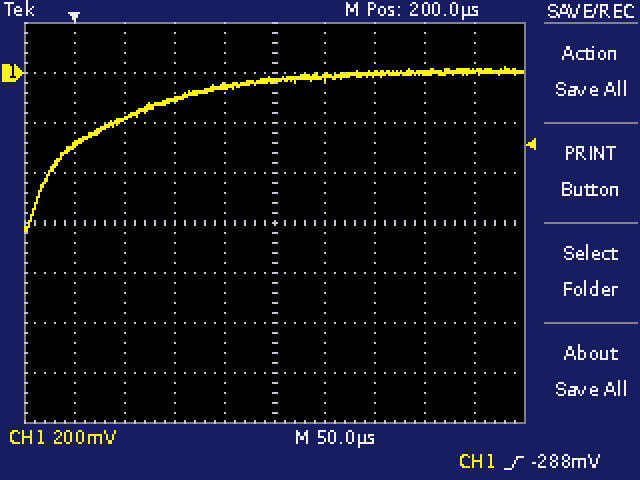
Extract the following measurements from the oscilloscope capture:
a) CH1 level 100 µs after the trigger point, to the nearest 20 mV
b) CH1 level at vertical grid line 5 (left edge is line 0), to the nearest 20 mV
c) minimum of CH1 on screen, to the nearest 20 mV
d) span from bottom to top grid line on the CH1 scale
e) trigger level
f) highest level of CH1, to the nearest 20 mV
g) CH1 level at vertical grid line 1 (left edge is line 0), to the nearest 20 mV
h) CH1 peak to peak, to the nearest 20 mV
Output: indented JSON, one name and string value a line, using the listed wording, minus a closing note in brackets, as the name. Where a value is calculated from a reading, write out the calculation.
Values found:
{
  "CH1 level 100 µs after the trigger point, to the nearest 20 mV": "-100 mV",
  "CH1 level at vertical grid line 5 (left edge is line 0), to the nearest 20 mV": "-40 mV",
  "minimum of CH1 on screen, to the nearest 20 mV": "-640 mV",
  "span from bottom to top grid line on the CH1 scale": "1.6 V",
  "trigger level": "-288 mV",
  "highest level of CH1, to the nearest 20 mV": "20 mV",
  "CH1 level at vertical grid line 1 (left edge is line 0), to the nearest 20 mV": "-280 mV",
  "CH1 peak to peak, to the nearest 20 mV": "20 mV − (-640 mV) = 660 mV"
}
